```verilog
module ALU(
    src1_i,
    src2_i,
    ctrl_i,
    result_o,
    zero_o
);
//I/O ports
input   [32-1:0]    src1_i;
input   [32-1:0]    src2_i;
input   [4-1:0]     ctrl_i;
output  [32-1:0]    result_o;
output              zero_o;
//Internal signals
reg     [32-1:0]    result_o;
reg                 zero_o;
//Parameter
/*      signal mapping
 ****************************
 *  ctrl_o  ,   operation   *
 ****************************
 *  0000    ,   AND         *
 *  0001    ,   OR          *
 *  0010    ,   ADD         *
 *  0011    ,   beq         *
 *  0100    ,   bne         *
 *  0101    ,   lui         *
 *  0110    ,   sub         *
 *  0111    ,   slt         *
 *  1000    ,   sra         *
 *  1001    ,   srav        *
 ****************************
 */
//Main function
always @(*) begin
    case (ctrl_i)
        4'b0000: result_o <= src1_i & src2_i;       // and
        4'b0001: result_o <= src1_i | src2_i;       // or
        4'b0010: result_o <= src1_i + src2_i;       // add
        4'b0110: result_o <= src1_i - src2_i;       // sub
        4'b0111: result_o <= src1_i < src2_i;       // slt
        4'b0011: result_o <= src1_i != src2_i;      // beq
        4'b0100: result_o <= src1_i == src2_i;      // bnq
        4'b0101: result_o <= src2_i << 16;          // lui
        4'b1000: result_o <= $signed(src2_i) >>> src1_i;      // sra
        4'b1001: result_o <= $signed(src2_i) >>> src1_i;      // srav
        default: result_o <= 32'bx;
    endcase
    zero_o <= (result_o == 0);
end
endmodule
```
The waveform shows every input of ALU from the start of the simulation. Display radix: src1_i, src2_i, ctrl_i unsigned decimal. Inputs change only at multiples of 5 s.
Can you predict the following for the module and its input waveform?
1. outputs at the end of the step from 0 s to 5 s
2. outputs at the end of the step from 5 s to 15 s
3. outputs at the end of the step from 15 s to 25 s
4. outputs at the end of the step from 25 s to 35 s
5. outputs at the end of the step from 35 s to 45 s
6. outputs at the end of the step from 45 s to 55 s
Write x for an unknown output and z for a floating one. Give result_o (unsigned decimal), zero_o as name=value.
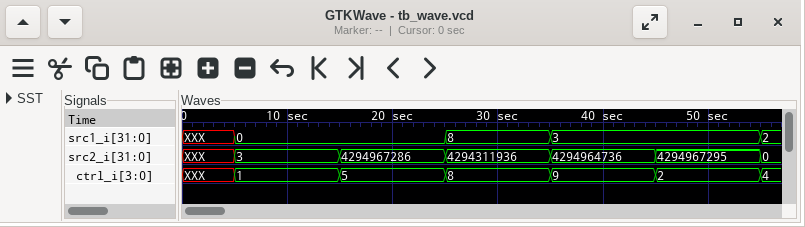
result_o=x, zero_o=x
result_o=3, zero_o=0
result_o=4294311936, zero_o=0
result_o=4294964736, zero_o=0
result_o=4294966976, zero_o=0
result_o=2, zero_o=0
